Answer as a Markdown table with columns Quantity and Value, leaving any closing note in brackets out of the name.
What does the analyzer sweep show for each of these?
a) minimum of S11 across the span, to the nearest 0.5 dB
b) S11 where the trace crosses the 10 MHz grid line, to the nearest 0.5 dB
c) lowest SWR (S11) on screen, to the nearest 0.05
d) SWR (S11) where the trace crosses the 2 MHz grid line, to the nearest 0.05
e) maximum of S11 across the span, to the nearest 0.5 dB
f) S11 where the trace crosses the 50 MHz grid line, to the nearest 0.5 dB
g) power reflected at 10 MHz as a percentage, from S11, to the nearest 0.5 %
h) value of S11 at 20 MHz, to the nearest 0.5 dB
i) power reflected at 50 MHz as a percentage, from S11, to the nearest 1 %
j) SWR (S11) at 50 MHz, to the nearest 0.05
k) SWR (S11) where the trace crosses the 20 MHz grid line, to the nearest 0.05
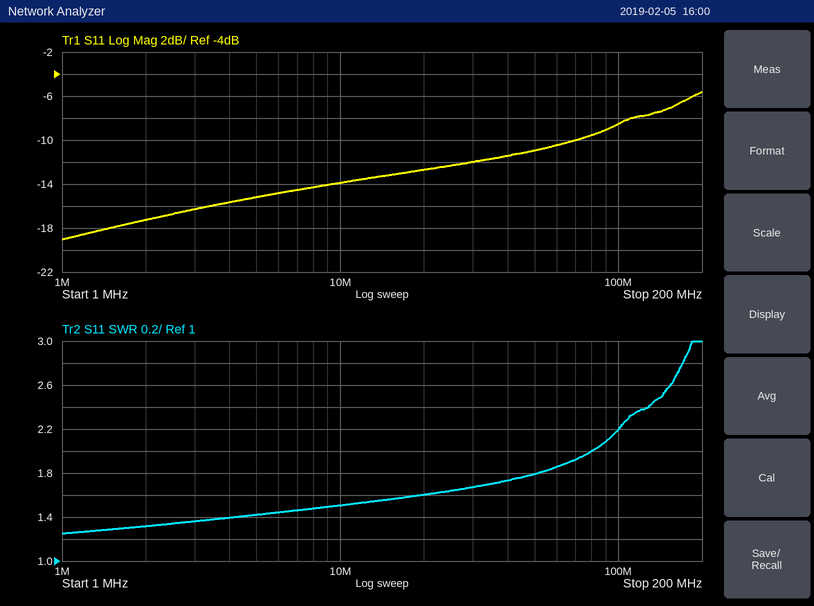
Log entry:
| Quantity | Value |
|---|---|
| minimum of S11 across the span, to the nearest 0.5 dB | -19.0 dB |
| S11 where the trace crosses the 10 MHz grid line, to the nearest 0.5 dB | -14.0 dB |
| lowest SWR (S11) on screen, to the nearest 0.05 | 1.25 |
| SWR (S11) where the trace crosses the 2 MHz grid line, to the nearest 0.05 | 1.30 |
| maximum of S11 across the span, to the nearest 0.5 dB | -5.5 dB |
| S11 where the trace crosses the 50 MHz grid line, to the nearest 0.5 dB | -11.0 dB |
| power reflected at 10 MHz as a percentage, from S11, to the nearest 0.5 % | 4.0 % |
| value of S11 at 20 MHz, to the nearest 0.5 dB | -12.5 dB |
| power reflected at 50 MHz as a percentage, from S11, to the nearest 1 % | 8 % |
| SWR (S11) at 50 MHz, to the nearest 0.05 | 1.80 |
| SWR (S11) where the trace crosses the 20 MHz grid line, to the nearest 0.05 | 1.60 |
